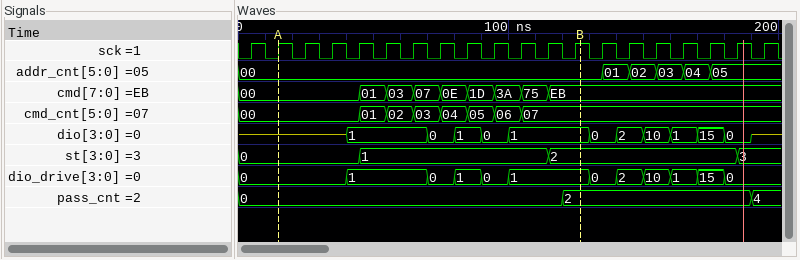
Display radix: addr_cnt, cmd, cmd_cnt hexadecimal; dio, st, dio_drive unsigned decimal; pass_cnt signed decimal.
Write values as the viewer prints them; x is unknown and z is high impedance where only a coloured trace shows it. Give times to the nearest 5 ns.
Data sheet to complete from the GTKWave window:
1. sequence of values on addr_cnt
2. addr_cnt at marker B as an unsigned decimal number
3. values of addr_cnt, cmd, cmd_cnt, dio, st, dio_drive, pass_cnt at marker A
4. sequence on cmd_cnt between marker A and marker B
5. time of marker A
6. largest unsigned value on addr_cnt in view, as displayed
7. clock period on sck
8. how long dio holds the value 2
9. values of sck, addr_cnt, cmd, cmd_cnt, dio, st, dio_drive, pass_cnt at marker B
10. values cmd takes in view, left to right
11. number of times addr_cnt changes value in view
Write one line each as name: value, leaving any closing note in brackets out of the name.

sequence of values on addr_cnt: 00, 01, 02, 03, 04, 05
addr_cnt at marker B as an unsigned decimal number: 0
values of addr_cnt, cmd, cmd_cnt, dio, st, dio_drive, pass_cnt at marker A: addr_cnt=00, cmd=00, cmd_cnt=00, dio=z, st=0, dio_drive=0, pass_cnt=0
sequence on cmd_cnt between marker A and marker B: 00, 01, 02, 03, 04, 05, 06, 07
time of marker A: 15 ns
largest unsigned value on addr_cnt in view, as displayed: 05
clock period on sck: 10 ns
how long dio holds the value 2: 10 ns
values of sck, addr_cnt, cmd, cmd_cnt, dio, st, dio_drive, pass_cnt at marker B: sck=1, addr_cnt=00, cmd=EB, cmd_cnt=07, dio=1, st=2, dio_drive=1, pass_cnt=2
values cmd takes in view, left to right: 00, 01, 03, 07, 0E, 1D, 3A, 75, EB
number of times addr_cnt changes value in view: 5
